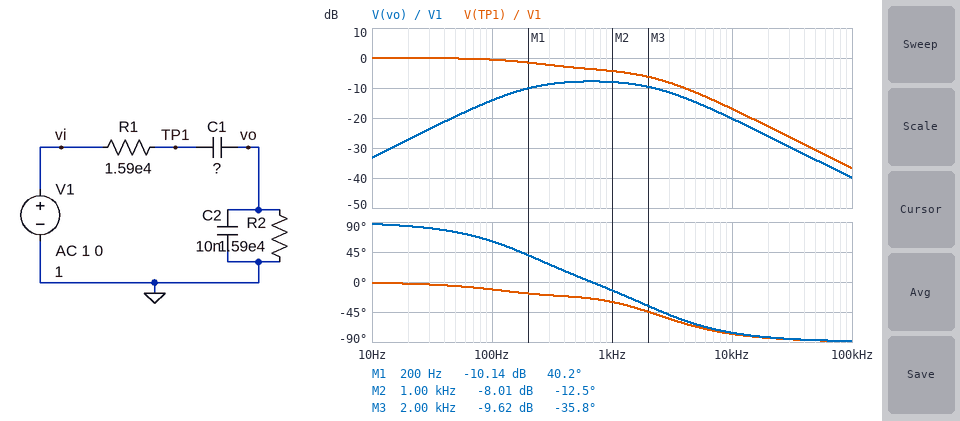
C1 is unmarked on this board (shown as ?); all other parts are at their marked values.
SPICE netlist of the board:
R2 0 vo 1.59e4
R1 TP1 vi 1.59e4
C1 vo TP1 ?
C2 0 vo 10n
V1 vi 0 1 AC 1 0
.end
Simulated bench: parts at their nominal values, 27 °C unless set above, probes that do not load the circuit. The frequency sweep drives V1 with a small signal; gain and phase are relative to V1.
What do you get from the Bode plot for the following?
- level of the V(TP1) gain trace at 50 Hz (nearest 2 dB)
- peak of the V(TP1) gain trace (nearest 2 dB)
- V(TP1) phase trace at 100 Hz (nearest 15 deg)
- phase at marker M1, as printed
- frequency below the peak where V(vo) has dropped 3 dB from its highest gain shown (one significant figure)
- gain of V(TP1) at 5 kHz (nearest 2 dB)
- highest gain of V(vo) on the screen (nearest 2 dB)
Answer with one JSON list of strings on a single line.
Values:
["0 dB", "0 dB", "-15 deg", "40.2 deg", "200 Hz", "-12 dB", "-8 dB"]
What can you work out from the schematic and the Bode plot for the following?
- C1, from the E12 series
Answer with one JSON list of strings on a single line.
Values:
["22 nF"]
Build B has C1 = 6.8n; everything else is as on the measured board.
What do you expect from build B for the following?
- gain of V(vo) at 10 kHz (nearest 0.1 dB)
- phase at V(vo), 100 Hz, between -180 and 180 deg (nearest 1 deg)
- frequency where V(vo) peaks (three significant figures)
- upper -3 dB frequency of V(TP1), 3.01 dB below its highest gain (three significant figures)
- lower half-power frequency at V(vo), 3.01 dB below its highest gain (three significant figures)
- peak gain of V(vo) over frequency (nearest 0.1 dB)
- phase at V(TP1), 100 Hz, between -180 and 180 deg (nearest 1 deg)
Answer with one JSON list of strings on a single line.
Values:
["-20.4 dB", "77 deg", "1.21 kHz", "1.92 kHz", "382 Hz", "-10.8 dB", "-4 deg"]
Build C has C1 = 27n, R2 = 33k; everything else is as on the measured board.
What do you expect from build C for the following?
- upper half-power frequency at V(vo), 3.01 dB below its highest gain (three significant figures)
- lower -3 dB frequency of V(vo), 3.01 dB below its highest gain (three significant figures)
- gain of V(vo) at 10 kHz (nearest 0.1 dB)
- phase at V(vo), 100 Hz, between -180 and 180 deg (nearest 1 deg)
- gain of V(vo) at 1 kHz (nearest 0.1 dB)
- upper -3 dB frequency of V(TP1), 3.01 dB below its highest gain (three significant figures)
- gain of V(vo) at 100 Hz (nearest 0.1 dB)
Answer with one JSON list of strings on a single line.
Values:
["1.95 kHz", "91.9 Hz", "-20.1 dB", "42 deg", "-6.1 dB", "853 Hz", "-8.0 dB"]
